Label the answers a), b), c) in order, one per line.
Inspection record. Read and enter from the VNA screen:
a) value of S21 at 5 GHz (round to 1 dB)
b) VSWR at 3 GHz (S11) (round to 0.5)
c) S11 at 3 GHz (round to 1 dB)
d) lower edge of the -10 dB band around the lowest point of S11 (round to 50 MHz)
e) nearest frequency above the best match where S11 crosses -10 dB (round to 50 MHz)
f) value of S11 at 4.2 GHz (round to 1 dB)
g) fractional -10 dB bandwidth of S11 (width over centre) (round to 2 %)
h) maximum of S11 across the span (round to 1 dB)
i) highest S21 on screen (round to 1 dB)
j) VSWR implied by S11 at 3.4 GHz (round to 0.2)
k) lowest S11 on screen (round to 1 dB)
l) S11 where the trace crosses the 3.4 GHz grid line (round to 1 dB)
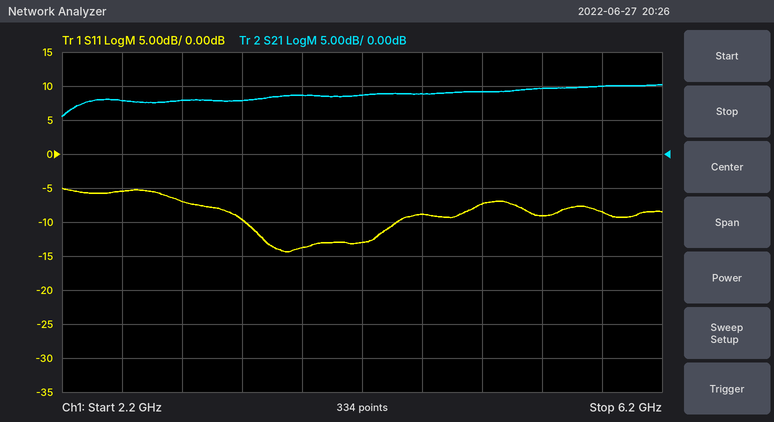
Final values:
a) 9 dB
b) 2.5
c) -7 dB
d) 3.40 GHz
e) 4.45 GHz
f) -13 dB
g) 26 %
h) -5 dB
i) 10 dB
j) 2.0
k) -14 dB
l) -10 dB
